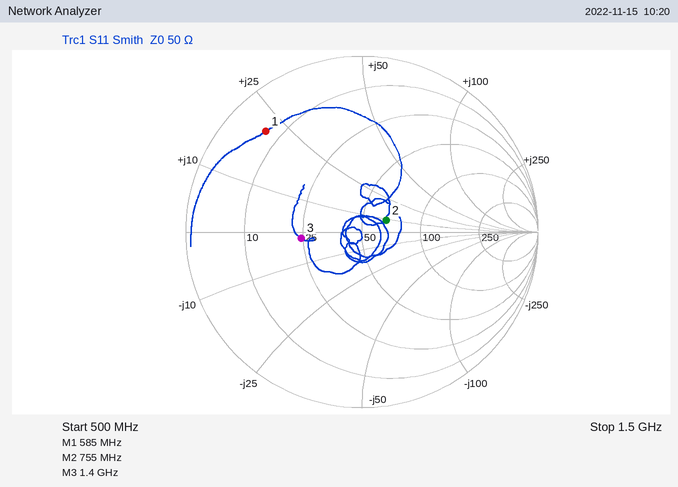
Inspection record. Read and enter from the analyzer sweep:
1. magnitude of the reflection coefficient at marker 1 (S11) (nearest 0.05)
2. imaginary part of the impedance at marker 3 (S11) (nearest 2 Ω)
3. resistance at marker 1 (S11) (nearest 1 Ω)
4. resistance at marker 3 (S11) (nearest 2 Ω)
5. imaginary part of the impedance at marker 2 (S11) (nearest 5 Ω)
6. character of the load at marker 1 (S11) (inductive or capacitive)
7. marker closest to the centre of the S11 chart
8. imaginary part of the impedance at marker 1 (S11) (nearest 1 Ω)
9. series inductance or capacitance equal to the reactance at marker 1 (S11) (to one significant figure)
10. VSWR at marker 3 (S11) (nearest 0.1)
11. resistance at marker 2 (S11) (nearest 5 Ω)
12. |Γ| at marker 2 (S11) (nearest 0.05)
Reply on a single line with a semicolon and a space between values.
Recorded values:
0.80; -2 Ω; 7 Ω; 24 Ω; +10 Ω; inductive; marker 2; +21 Ω; 6 nH; 2.1; 65 Ω; 0.15
